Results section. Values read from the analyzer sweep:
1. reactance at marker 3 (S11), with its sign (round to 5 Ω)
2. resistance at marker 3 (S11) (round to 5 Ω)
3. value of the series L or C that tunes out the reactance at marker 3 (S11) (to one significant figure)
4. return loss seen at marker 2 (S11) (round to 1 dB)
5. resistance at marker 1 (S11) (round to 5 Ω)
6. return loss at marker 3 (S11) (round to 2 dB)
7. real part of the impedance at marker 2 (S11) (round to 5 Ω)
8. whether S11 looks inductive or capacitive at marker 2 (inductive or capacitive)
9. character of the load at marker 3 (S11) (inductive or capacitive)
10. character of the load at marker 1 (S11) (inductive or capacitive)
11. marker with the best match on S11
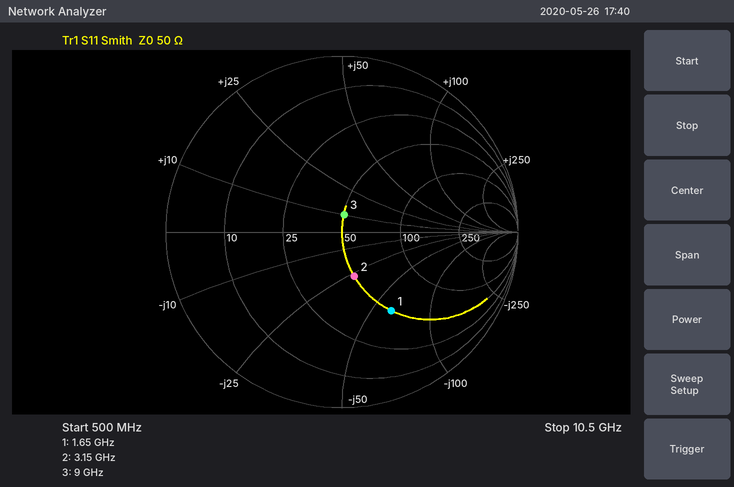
+10 Ω
50 Ω
2 pF
12 dB
50 Ω
20 dB
50 Ω
capacitive
inductive
capacitive
marker 3
